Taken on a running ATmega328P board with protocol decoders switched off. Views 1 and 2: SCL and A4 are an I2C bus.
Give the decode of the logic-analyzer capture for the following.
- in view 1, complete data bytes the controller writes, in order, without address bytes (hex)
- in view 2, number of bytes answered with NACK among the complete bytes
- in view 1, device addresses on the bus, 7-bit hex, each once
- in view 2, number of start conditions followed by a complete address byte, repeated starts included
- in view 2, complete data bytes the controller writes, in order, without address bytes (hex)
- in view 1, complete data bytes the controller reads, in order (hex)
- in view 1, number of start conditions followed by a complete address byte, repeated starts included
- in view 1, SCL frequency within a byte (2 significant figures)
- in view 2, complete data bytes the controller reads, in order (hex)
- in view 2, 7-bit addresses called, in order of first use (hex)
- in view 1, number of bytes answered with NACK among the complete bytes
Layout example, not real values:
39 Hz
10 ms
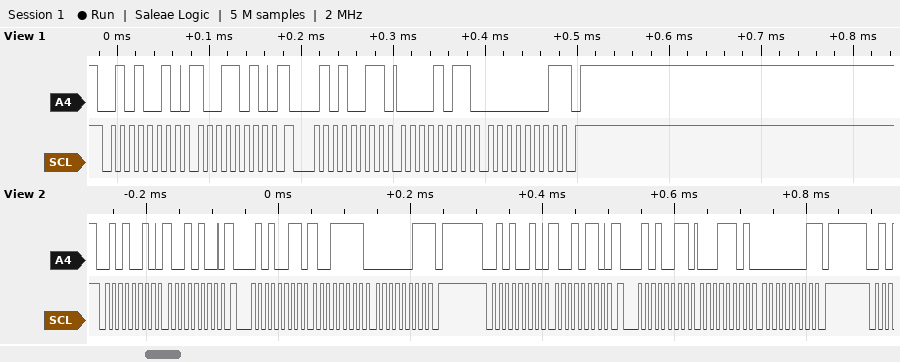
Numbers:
9A
2
0x29
4
94 96
0B 01
2
100 kHz
9F 03 1D 01
0x29
1
